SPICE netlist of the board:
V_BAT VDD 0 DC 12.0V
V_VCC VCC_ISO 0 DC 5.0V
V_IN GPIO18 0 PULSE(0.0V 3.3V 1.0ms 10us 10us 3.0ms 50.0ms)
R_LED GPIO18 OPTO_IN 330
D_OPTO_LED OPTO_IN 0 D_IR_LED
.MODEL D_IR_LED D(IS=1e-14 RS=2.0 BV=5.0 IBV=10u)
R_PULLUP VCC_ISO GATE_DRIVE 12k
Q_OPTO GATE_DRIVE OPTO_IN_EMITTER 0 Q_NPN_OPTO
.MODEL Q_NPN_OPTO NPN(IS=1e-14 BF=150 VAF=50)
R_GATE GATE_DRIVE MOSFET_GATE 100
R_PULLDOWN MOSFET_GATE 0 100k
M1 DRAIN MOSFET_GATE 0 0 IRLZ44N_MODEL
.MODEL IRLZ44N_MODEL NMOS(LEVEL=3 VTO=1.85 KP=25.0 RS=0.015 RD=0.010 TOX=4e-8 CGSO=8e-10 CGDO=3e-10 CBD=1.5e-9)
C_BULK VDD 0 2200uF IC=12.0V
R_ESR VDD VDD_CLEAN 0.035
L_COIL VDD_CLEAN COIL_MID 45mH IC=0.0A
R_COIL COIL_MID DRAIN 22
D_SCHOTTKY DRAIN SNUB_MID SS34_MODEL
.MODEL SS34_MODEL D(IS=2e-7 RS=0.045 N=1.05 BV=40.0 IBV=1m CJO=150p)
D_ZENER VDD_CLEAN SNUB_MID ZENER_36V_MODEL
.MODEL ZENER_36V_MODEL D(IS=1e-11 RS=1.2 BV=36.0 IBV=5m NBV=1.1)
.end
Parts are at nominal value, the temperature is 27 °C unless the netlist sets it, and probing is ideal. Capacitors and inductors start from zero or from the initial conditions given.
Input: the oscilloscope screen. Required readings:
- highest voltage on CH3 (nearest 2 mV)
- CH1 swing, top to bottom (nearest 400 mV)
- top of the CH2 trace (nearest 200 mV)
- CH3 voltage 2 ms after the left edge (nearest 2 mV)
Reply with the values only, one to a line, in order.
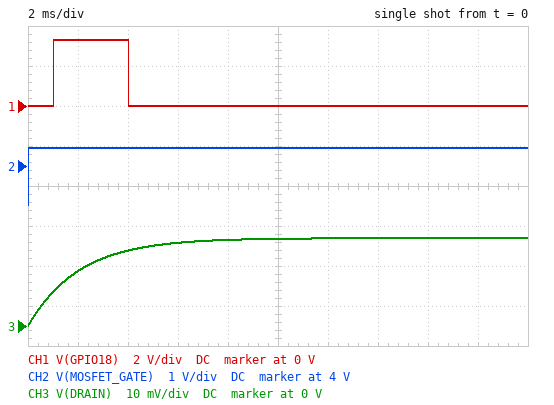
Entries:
22 mV
3.2 V
4.4 V
14 mV
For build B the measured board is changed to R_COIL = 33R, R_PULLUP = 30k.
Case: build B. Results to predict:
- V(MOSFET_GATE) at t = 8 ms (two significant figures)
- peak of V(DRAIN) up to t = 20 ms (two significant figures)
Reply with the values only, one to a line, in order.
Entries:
3.8 V
16 mV
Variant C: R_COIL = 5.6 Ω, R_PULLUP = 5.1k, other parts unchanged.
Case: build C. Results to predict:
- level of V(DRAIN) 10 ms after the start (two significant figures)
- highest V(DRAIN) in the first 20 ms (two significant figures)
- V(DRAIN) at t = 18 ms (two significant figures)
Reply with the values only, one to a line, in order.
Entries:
59 mV
76 mV
74 mV
